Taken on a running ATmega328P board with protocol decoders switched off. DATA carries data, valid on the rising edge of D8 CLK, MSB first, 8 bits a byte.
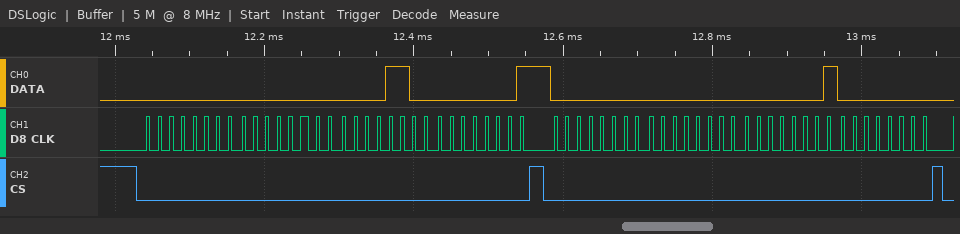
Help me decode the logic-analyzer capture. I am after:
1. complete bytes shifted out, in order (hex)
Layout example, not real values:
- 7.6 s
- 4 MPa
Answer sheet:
- 0x00 0x00 0x0C 0x01 0x00 0x00 0x01 0x00
